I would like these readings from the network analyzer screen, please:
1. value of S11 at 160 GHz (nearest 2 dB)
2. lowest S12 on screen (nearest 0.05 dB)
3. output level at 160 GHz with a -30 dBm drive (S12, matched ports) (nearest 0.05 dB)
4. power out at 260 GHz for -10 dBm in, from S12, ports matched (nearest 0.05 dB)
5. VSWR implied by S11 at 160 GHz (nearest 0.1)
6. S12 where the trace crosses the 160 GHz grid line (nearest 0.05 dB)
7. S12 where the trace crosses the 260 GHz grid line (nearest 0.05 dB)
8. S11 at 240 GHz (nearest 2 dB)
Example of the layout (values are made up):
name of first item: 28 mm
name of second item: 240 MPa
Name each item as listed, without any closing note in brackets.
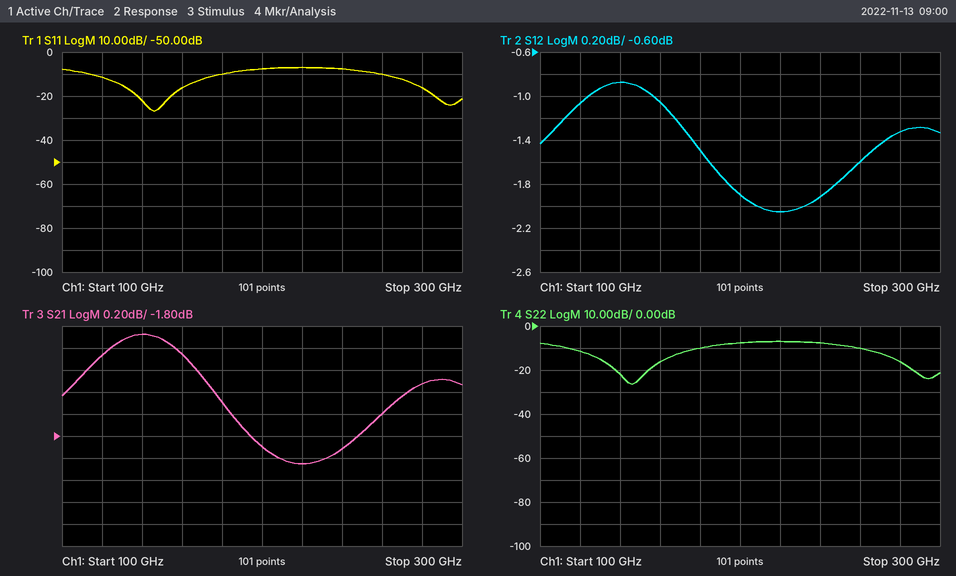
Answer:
value of S11 at 160 GHz: -16 dB
lowest S12 on screen: -2.05 dB
output level at 160 GHz with a -30 dBm drive (S12, matched ports): -31.05 dBm
power out at 260 GHz for -10 dBm in, from S12, ports matched: -11.60 dBm
VSWR implied by S11 at 160 GHz: 1.4
S12 where the trace crosses the 160 GHz grid line: -1.05 dB
S12 where the trace crosses the 260 GHz grid line: -1.60 dB
S11 at 240 GHz: -8 dB
